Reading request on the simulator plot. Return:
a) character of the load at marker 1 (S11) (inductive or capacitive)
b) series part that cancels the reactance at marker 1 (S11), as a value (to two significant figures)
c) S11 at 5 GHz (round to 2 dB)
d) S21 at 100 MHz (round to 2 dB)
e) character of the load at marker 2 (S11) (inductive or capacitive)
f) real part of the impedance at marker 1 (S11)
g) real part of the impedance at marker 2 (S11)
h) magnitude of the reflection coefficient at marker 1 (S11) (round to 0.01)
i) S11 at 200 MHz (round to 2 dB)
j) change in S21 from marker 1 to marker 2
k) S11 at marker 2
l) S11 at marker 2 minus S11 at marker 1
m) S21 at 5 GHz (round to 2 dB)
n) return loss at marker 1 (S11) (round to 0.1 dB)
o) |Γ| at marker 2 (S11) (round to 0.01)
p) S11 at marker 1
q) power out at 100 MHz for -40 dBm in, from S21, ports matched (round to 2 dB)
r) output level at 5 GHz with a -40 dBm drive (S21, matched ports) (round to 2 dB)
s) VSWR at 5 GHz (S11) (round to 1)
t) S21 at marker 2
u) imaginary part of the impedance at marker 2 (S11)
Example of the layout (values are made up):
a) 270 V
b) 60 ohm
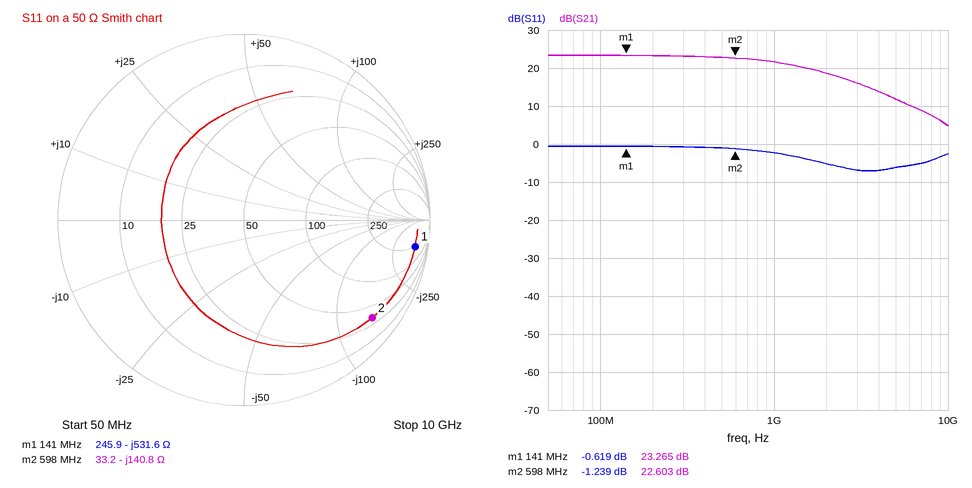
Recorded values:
a) capacitive
b) 600 nH
c) -6 dB
d) 24 dB
e) capacitive
f) 245.9 Ω
g) 33.2 Ω
h) 0.93
i) 0 dB
j) -0.662 dB
k) -1.239 dB
l) -0.620 dB
m) 12 dB
n) 0.6 dB
o) 0.87
p) -0.619 dB
q) -16 dBm
r) -28 dBm
s) 3
t) 22.603 dB
u) -140.8 Ω
